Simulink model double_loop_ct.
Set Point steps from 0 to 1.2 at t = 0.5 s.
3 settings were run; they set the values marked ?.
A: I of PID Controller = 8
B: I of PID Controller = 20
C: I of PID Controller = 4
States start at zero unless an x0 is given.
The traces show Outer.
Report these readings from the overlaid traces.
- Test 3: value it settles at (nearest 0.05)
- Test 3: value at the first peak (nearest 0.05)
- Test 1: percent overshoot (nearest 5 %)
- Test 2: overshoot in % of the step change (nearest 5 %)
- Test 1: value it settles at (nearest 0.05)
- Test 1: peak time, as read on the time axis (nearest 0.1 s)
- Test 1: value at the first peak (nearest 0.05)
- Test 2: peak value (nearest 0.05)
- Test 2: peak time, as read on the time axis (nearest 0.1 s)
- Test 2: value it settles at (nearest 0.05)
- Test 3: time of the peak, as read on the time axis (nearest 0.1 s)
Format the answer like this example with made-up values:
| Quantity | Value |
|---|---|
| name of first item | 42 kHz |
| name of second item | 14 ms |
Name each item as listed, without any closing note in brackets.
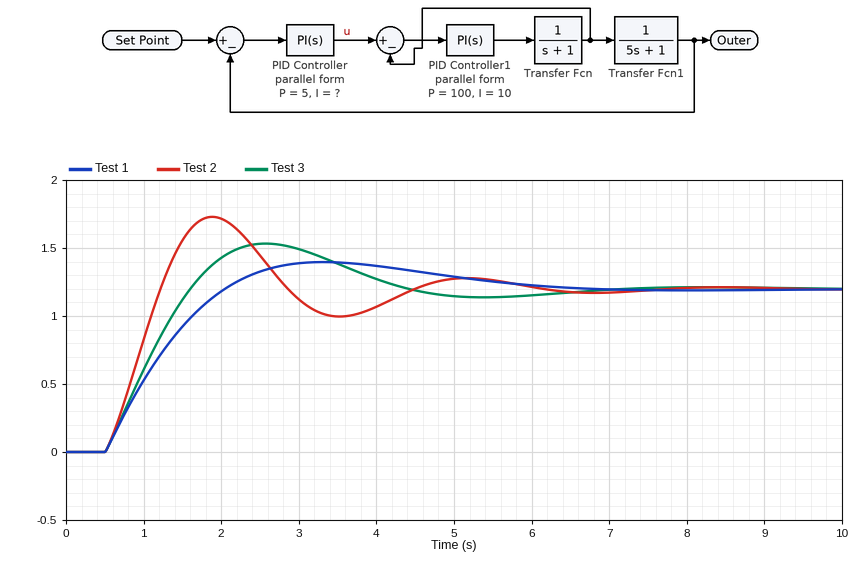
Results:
| Quantity | Value |
|---|---|
| Test 3: value it settles at | 1.20 |
| Test 3: value at the first peak | 1.55 |
| Test 1: percent overshoot | 15 % |
| Test 2: overshoot in % of the step change | 45 % |
| Test 1: value it settles at | 1.20 |
| Test 1: peak time, as read on the time axis | 3.3 s |
| Test 1: value at the first peak | 1.40 |
| Test 2: peak value | 1.75 |
| Test 2: peak time, as read on the time axis | 1.9 s |
| Test 2: value it settles at | 1.20 |
| Test 3: time of the peak, as read on the time axis | 2.6 s |
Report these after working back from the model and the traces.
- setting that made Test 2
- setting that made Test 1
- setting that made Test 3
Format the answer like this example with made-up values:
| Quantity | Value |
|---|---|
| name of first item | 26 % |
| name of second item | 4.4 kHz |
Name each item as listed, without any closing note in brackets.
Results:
| Quantity | Value |
|---|---|
| setting that made Test 2 | B |
| setting that made Test 1 | C |
| setting that made Test 3 | A |
